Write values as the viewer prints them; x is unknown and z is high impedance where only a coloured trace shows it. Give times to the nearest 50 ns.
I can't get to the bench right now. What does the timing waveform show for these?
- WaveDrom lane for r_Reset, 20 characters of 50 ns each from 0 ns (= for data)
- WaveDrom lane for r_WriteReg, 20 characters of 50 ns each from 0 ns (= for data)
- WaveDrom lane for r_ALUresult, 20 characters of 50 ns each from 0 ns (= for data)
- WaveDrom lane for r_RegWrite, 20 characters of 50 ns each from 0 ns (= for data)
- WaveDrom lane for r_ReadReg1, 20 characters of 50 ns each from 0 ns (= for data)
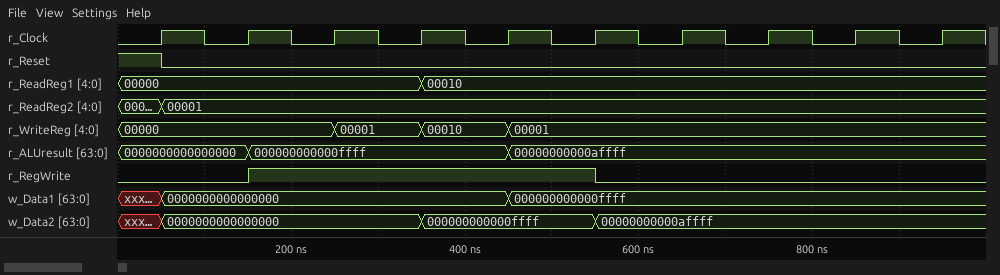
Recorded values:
{name: 'r_Reset', wave: '10..................'}
{name: 'r_WriteReg', wave: '=....=.=.=..........', data: '00000 00001 00010 00001'}
{name: 'r_ALUresult', wave: '=..=.....=..........', data: '0000000000000000 000000000000ffff 00000000000affff'}
{name: 'r_RegWrite', wave: '0..1.......0........'}
{name: 'r_ReadReg1', wave: '=......=............', data: '00000 00010'}
